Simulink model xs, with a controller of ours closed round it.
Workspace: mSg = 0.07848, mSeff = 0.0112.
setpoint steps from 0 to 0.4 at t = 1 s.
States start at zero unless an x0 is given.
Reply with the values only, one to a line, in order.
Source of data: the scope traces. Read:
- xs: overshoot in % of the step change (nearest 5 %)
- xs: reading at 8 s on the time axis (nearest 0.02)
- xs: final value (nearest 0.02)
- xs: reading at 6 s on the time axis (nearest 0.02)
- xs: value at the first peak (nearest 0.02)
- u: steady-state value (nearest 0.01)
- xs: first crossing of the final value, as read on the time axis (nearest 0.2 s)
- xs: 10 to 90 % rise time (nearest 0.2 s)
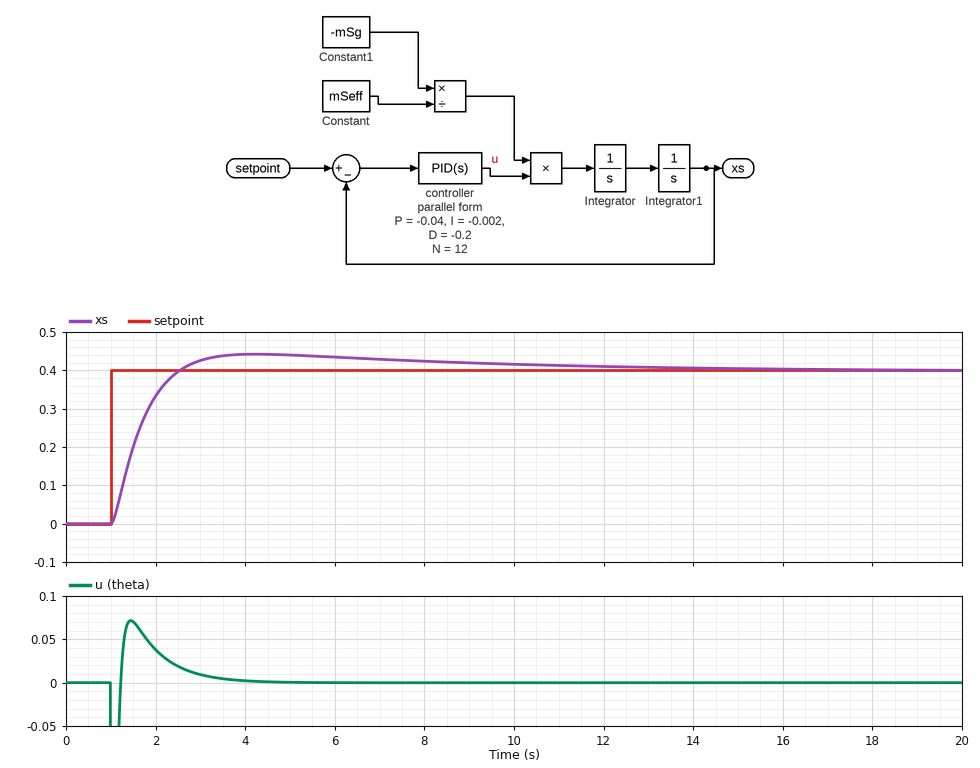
10 %
0.42
0.40
0.44
0.44
0.00
2.6 s
1.0 s
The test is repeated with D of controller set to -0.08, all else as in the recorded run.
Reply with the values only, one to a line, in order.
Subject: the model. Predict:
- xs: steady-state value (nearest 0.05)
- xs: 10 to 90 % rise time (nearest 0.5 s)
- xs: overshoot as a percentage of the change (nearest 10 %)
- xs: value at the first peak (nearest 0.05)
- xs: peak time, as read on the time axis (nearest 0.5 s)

0.40
1.5 s
30 %
0.55
5.5 s
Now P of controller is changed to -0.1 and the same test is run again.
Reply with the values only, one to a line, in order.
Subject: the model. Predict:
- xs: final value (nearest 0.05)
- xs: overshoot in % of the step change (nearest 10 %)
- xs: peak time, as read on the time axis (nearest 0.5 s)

0.40
20 %
3.5 s
